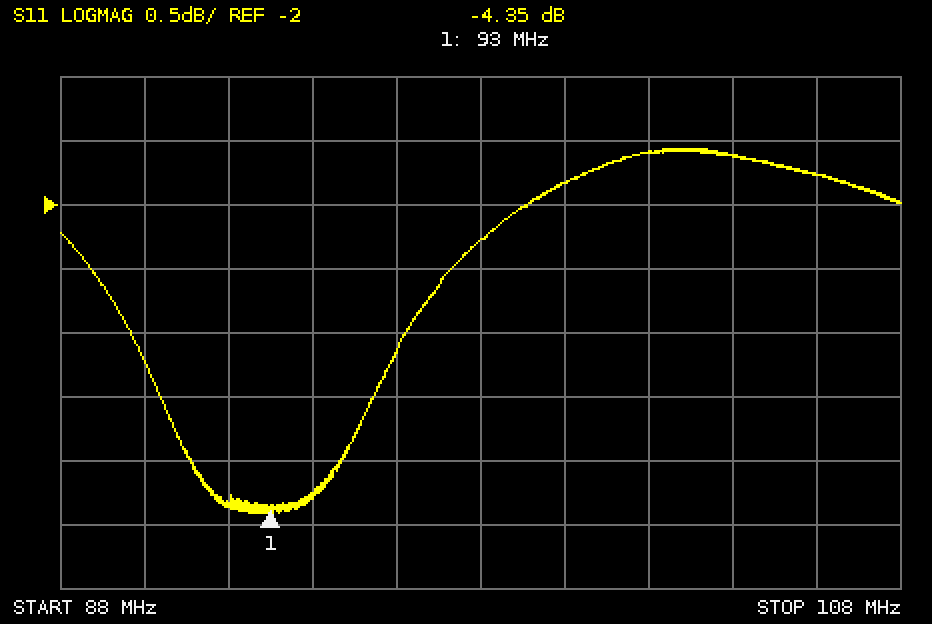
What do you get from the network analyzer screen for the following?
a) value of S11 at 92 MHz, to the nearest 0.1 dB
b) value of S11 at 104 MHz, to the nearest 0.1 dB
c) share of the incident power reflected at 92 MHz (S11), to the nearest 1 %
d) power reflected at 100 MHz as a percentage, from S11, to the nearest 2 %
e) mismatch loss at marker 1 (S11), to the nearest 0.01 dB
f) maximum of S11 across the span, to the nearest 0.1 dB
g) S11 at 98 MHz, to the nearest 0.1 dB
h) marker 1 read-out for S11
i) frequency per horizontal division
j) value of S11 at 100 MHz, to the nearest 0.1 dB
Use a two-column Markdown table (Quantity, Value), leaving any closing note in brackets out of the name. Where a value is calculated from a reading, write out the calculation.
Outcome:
| Quantity | Value |
|---|---|
| value of S11 at 92 MHz, to the nearest 0.1 dB | -4.3 dB |
| value of S11 at 104 MHz, to the nearest 0.1 dB | -1.6 dB |
| share of the incident power reflected at 92 MHz (S11), to the nearest 1 % | 10^(-4.3/10) ≈ 37 % |
| power reflected at 100 MHz as a percentage, from S11, to the nearest 2 % | 10^(-1.8/10) ≈ 66 % |
| mismatch loss at marker 1 (S11), to the nearest 0.01 dB | −10 log10(1 − 10^(-4.35/10)) ≈ 1.99 dB |
| maximum of S11 across the span, to the nearest 0.1 dB | -1.6 dB |
| S11 at 98 MHz, to the nearest 0.1 dB | -2.3 dB |
| marker 1 read-out for S11 | -4.35 dB |
| frequency per horizontal division | 2 MHz |
| value of S11 at 100 MHz, to the nearest 0.1 dB | -1.8 dB |
